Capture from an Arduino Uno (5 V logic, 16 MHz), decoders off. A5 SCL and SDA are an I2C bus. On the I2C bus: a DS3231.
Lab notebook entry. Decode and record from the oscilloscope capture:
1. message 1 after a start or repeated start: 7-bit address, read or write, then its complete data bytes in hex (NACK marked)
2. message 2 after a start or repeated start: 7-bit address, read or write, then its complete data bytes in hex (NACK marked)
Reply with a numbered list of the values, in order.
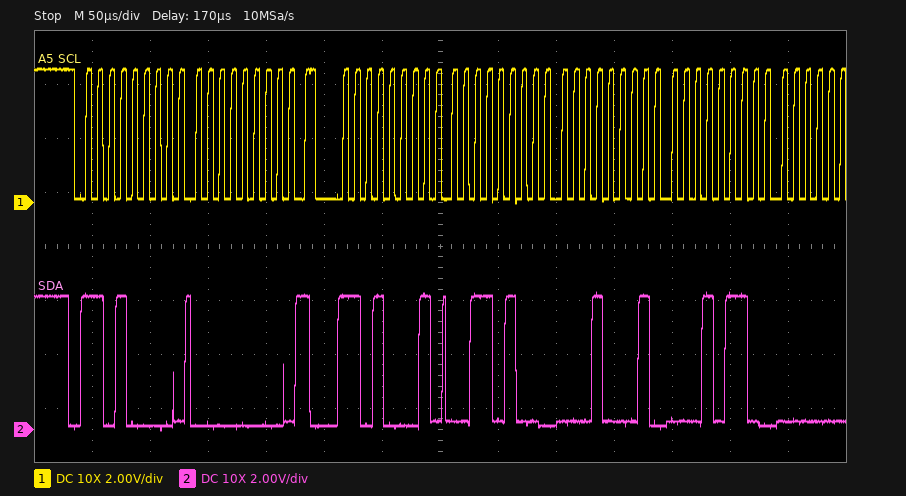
1. 0x68 write: 00
2. 0x68 read: 34 11 16
